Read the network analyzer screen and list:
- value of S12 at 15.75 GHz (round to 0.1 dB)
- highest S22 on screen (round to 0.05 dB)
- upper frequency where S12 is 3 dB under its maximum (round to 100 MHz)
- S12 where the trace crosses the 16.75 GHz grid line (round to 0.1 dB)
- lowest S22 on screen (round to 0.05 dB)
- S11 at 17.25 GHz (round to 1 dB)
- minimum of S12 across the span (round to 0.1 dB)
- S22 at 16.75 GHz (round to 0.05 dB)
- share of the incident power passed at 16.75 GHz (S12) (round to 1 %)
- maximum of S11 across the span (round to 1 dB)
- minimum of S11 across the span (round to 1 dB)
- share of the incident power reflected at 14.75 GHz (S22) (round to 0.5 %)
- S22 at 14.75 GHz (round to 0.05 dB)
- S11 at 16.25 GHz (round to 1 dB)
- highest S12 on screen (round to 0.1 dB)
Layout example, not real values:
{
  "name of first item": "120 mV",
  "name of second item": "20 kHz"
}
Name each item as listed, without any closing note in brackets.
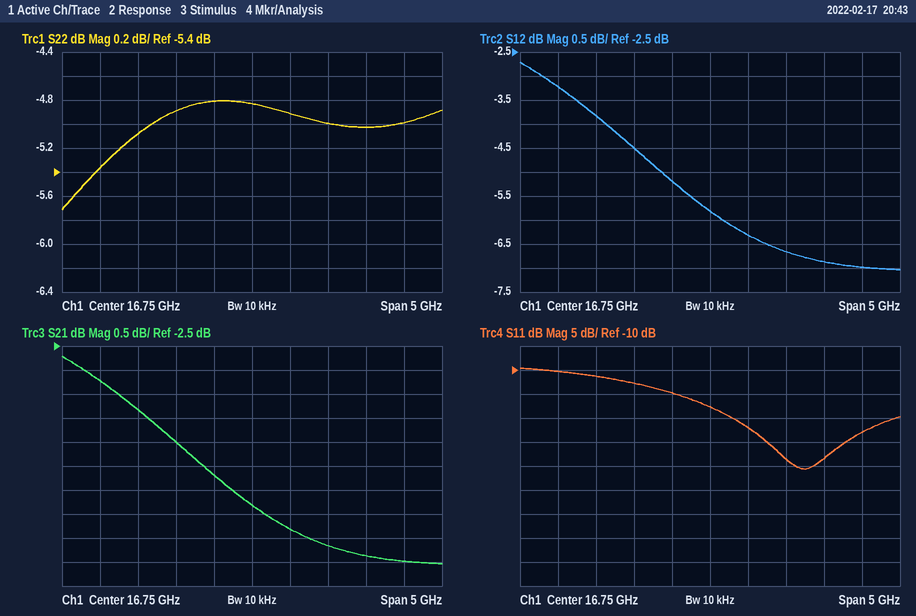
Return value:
{
  "value of S12 at 15.75 GHz": "-4.5 dB",
  "highest S22 on screen": "-4.80 dB",
  "upper frequency where S12 is 3 dB under its maximum": "16.7 GHz",
  "S12 where the trace crosses the 16.75 GHz grid line": "-5.8 dB",
  "lowest S22 on screen": "-5.70 dB",
  "S11 at 17.25 GHz": "-22 dB",
  "minimum of S12 across the span": "-7.0 dB",
  "S22 at 16.75 GHz": "-4.85 dB",
  "share of the incident power passed at 16.75 GHz (S12)": "26 %",
  "maximum of S11 across the span": "-10 dB",
  "minimum of S11 across the span": "-31 dB",
  "share of the incident power reflected at 14.75 GHz (S22)": "29.0 %",
  "S22 at 14.75 GHz": "-5.35 dB",
  "S11 at 16.25 GHz": "-15 dB",
  "highest S12 on screen": "-2.7 dB"
}
